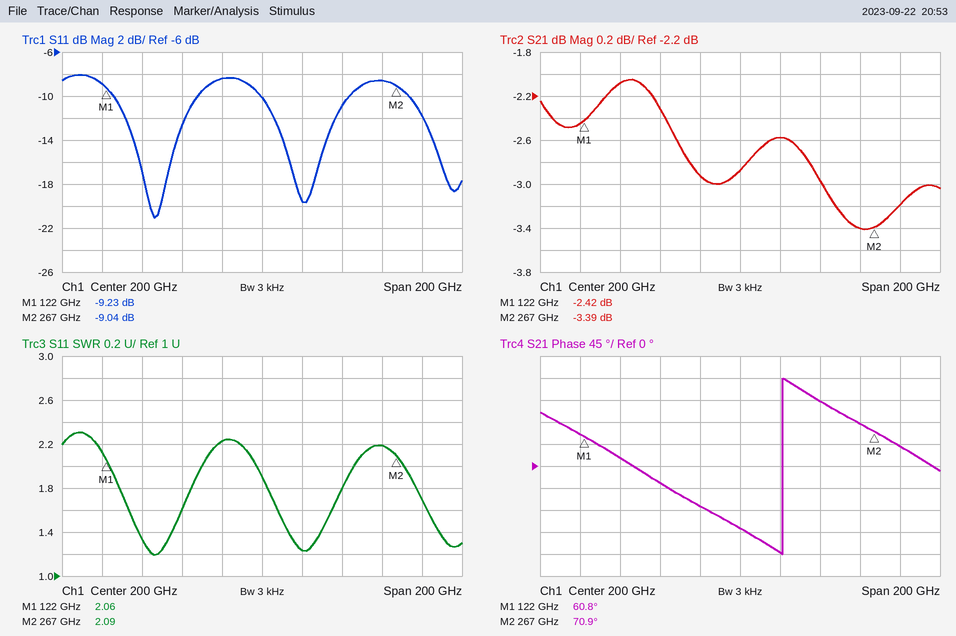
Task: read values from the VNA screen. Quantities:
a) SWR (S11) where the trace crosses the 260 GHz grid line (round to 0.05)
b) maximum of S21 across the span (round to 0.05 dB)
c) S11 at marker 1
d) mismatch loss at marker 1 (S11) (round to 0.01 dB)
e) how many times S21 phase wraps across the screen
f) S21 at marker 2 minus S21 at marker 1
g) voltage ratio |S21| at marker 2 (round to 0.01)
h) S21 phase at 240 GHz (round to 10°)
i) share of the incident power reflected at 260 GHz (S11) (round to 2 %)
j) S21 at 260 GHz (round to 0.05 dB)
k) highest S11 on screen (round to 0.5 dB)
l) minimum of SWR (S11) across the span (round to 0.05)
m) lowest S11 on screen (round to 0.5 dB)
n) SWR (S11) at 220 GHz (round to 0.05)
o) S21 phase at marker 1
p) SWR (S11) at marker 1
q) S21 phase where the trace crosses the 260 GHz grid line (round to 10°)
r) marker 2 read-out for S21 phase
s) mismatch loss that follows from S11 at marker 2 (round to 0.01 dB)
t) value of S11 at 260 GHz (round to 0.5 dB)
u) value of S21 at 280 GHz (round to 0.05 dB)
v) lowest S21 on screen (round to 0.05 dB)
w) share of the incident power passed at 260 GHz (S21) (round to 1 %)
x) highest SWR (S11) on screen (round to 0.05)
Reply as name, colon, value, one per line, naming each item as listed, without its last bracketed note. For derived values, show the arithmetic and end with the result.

SWR (S11) where the trace crosses the 260 GHz grid line: 2.20
maximum of S21 across the span: -2.05 dB
S11 at marker 1: -9.23 dB
mismatch loss at marker 1 (S11): −10 log10(1 − 10^(-9.23/10)) ≈ 0.55 dB
how many times S21 phase wraps across the screen: 1
S21 at marker 2 minus S21 at marker 1: -3.39 − (-2.42) = -0.97 dB
voltage ratio |S21| at marker 2: 10^(-3.39/20) ≈ 0.68
S21 phase at 240 GHz: 130°
share of the incident power reflected at 260 GHz (S11): 10^(-8.5/10) ≈ 14 %
S21 at 260 GHz: -3.40 dB
highest S11 on screen: -8.0 dB
minimum of SWR (S11) across the span: 1.20
lowest S11 on screen: -21.0 dB
SWR (S11) at 220 GHz: 1.25
S21 phase at marker 1: 60.8°
SWR (S11) at marker 1: 2.06
S21 phase where the trace crosses the 260 GHz grid line: 90°
marker 2 read-out for S21 phase: 70.9°
mismatch loss that follows from S11 at marker 2: −10 log10(1 − 10^(-9.04/10)) ≈ 0.58 dB
value of S11 at 260 GHz: -8.5 dB
value of S21 at 280 GHz: -3.20 dB
lowest S21 on screen: -3.40 dB
share of the incident power passed at 260 GHz (S21): 10^(-3.4/10) ≈ 46 %
highest SWR (S11) on screen: 2.30
